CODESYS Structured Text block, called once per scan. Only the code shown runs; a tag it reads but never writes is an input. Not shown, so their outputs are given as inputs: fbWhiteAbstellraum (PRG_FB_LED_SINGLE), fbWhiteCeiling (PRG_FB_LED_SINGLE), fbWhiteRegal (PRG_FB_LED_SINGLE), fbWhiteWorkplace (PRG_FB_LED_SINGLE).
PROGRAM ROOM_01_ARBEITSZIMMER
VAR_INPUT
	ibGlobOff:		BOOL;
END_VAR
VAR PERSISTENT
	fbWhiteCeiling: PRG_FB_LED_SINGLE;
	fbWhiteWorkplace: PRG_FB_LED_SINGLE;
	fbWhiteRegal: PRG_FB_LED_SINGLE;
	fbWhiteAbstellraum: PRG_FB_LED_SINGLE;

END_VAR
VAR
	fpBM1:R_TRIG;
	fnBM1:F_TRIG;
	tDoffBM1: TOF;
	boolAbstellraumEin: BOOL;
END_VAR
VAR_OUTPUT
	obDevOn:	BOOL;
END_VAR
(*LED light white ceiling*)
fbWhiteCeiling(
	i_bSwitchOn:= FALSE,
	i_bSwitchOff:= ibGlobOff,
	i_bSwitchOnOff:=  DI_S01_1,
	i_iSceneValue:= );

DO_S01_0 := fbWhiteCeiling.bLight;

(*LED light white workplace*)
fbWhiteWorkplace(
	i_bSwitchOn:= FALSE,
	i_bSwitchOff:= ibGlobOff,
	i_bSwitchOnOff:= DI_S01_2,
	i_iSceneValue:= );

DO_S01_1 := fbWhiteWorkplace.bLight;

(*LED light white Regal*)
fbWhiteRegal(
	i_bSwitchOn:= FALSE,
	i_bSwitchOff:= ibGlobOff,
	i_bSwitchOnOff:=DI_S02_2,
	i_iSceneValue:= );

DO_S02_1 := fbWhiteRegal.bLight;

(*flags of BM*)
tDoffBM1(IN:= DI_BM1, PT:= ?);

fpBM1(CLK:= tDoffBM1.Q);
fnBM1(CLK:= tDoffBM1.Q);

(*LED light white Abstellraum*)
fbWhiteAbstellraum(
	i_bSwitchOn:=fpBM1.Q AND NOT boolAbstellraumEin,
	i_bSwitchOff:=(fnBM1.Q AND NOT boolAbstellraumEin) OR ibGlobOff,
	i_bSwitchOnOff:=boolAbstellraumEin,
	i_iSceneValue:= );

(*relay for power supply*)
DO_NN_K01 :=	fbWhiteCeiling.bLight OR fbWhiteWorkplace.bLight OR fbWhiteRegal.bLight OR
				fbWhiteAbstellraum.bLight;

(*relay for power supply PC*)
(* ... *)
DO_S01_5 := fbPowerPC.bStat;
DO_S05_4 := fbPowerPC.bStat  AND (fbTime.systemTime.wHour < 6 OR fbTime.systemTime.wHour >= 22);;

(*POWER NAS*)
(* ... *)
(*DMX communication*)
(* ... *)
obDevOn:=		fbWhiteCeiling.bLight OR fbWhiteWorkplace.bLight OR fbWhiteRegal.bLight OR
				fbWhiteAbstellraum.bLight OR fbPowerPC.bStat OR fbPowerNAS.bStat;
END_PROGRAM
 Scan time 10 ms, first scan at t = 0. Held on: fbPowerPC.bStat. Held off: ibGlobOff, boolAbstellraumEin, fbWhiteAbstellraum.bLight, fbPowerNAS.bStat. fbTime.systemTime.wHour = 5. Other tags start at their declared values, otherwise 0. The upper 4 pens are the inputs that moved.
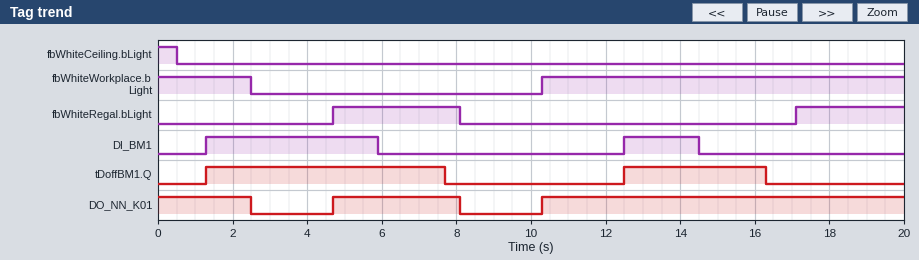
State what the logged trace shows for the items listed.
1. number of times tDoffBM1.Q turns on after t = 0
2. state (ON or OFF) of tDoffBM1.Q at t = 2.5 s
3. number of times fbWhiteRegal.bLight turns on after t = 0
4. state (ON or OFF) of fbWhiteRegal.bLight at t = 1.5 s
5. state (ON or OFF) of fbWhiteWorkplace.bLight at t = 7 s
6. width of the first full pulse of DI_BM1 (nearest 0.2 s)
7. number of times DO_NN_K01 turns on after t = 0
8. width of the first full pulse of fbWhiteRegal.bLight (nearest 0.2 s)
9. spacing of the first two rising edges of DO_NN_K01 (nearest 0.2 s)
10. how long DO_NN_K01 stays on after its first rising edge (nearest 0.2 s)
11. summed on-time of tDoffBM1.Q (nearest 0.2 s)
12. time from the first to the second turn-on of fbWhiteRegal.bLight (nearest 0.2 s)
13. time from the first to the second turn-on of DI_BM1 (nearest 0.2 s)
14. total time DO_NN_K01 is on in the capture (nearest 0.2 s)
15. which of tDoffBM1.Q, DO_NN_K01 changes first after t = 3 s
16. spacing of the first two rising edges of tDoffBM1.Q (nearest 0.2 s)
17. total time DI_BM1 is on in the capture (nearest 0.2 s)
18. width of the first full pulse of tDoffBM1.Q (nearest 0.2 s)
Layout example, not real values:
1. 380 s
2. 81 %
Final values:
1. 2
2. ON
3. 2
4. OFF
5. OFF
6. 4.6 s
7. 2
8. 3.4 s
9. 5.6 s
10. 3.4 s
11. 10.2 s
12. 12.4 s
13. 11.2 s
14. 15.6 s
15. DO_NN_K01
16. 11.2 s
17. 6.6 s
18. 6.4 s
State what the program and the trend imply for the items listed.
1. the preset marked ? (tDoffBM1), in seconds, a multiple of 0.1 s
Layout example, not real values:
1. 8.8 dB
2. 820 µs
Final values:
1. 1.8 s
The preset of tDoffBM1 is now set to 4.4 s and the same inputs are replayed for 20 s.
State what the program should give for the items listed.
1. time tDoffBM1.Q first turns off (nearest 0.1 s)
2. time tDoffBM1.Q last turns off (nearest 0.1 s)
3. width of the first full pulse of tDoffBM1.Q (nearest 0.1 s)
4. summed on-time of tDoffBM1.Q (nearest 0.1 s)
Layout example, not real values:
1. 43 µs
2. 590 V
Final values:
1. 10.3 s
2. 18.9 s
3. 9.0 s
4. 15.4 s
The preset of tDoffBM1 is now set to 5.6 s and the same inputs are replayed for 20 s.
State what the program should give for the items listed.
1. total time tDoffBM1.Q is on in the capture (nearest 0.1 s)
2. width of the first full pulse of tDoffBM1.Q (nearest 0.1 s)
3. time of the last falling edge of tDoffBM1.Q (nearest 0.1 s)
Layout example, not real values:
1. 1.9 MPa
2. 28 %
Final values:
1. 17.7 s
2. 10.2 s
3. 11.5 s
